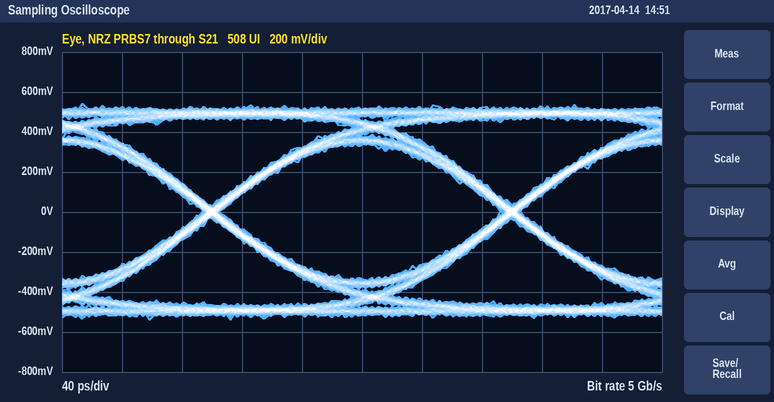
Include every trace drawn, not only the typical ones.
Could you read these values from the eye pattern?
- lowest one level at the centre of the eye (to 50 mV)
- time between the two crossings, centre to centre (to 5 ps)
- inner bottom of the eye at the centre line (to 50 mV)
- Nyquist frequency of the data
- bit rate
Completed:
350 mV
200 ps
-350 mV
2.5 GHz
5 Gb/s
